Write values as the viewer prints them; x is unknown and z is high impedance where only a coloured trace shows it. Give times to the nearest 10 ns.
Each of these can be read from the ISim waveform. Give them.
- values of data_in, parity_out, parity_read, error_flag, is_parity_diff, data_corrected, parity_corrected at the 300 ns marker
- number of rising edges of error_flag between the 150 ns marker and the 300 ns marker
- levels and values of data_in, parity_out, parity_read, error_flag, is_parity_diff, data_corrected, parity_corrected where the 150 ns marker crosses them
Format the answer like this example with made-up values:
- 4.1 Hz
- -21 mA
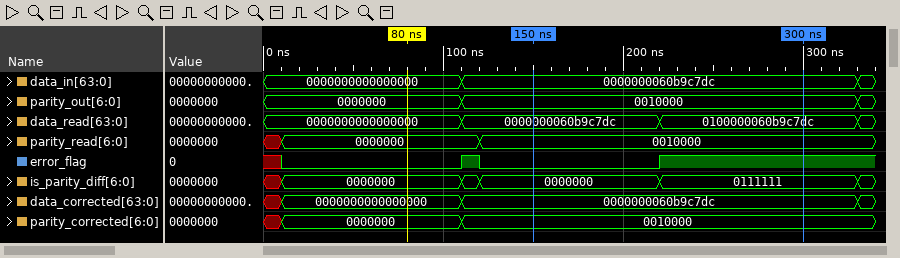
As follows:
- data_in=0000000060b9c7dc, parity_out=0010000, parity_read=0010000, error_flag=1, is_parity_diff=0111111, data_corrected=0000000060b9c7dc, parity_corrected=0010000
- 1
- data_in=0000000060b9c7dc, parity_out=0010000, parity_read=0010000, error_flag=0, is_parity_diff=0000000, data_corrected=0000000060b9c7dc, parity_corrected=0010000
